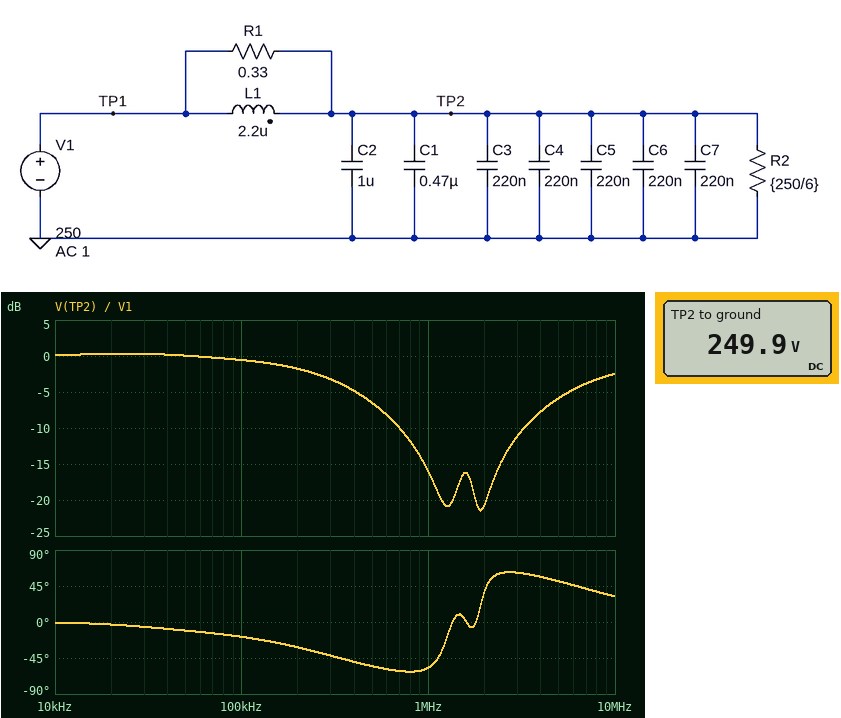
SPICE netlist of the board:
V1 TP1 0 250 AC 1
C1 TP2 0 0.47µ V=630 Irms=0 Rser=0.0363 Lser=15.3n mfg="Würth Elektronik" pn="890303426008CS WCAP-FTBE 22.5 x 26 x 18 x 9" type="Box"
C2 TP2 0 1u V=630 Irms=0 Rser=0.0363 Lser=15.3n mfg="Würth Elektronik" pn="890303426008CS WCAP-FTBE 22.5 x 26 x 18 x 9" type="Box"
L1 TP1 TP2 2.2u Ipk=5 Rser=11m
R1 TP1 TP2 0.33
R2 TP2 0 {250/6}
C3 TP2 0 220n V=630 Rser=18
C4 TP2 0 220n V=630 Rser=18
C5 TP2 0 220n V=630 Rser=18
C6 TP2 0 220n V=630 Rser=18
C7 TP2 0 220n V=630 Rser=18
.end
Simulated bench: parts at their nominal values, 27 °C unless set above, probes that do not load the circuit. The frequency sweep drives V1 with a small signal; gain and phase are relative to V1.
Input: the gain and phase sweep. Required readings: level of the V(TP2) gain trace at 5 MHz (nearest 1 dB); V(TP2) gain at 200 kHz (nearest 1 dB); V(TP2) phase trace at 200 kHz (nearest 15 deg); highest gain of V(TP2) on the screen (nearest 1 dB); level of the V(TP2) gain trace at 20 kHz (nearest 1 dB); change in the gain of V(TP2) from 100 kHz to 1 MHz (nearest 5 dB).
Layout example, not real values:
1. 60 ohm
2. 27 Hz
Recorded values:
1. -6 dB
2. -2 dB
3. -30 deg
4. 0 dB
5. 0 dB
6. -15 dB
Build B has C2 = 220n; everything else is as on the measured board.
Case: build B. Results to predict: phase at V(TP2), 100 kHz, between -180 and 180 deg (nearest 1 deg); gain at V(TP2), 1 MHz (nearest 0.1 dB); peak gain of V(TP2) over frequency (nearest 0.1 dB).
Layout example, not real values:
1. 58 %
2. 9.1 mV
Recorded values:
1. -10 deg
2. -7.1 dB
3. 0.2 dB
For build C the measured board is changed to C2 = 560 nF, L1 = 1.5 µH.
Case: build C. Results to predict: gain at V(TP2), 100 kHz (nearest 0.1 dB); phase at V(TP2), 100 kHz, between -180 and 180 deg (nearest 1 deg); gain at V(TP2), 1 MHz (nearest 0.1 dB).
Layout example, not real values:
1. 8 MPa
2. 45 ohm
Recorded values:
1. -0.3 dB
2. -14 deg
3. -10.6 dB
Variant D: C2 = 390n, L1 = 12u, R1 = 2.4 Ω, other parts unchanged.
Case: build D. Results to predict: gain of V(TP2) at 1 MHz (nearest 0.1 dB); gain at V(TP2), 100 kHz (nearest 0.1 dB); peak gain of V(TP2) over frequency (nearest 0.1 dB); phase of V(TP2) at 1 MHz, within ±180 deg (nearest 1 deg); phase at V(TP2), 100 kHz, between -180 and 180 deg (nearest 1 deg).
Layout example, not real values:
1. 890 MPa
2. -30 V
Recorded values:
1. -25.0 dB
2. -5.8 dB
3. 1.4 dB
4. -79 deg
5. -54 deg
